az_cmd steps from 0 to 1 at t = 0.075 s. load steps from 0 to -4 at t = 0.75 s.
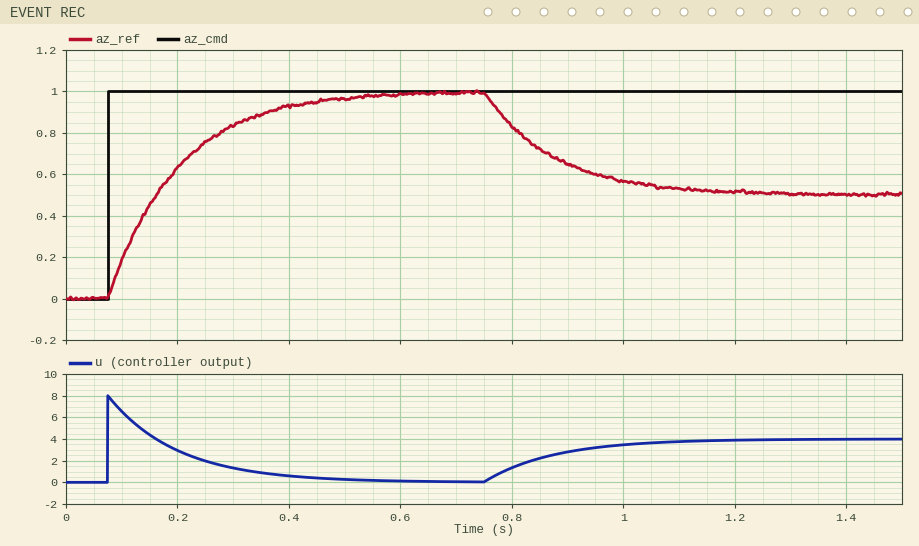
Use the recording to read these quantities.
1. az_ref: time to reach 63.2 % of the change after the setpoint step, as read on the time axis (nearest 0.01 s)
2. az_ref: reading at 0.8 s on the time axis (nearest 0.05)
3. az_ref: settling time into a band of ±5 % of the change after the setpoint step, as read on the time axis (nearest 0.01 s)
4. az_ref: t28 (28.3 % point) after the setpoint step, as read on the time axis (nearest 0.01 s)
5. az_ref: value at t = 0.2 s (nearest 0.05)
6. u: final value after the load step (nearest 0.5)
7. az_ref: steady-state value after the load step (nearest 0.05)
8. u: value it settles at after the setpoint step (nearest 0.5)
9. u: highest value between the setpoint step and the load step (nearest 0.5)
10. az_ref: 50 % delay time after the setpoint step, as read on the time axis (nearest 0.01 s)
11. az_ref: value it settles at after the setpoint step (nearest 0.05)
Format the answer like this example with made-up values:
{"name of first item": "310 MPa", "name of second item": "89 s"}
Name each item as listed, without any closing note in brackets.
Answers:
{"az_ref: time to reach 63.2 % of the change after the setpoint step, as read on the time axis": "0.20 s", "az_ref: reading at 0.8 s on the time axis": "0.85", "az_ref: settling time into a band of ±5 % of the change after the setpoint step, as read on the time axis": "0.45 s", "az_ref: t28 (28.3 % point) after the setpoint step, as read on the time axis": "0.12 s", "az_ref: value at t = 0.2 s": "0.65", "u: final value after the load step": "4.0", "az_ref: steady-state value after the load step": "0.50", "u: value it settles at after the setpoint step": "0.0", "u: highest value between the setpoint step and the load step": "8.0", "az_ref: 50 % delay time after the setpoint step, as read on the time axis": "0.16 s", "az_ref: value it settles at after the setpoint step": "1.00"}
